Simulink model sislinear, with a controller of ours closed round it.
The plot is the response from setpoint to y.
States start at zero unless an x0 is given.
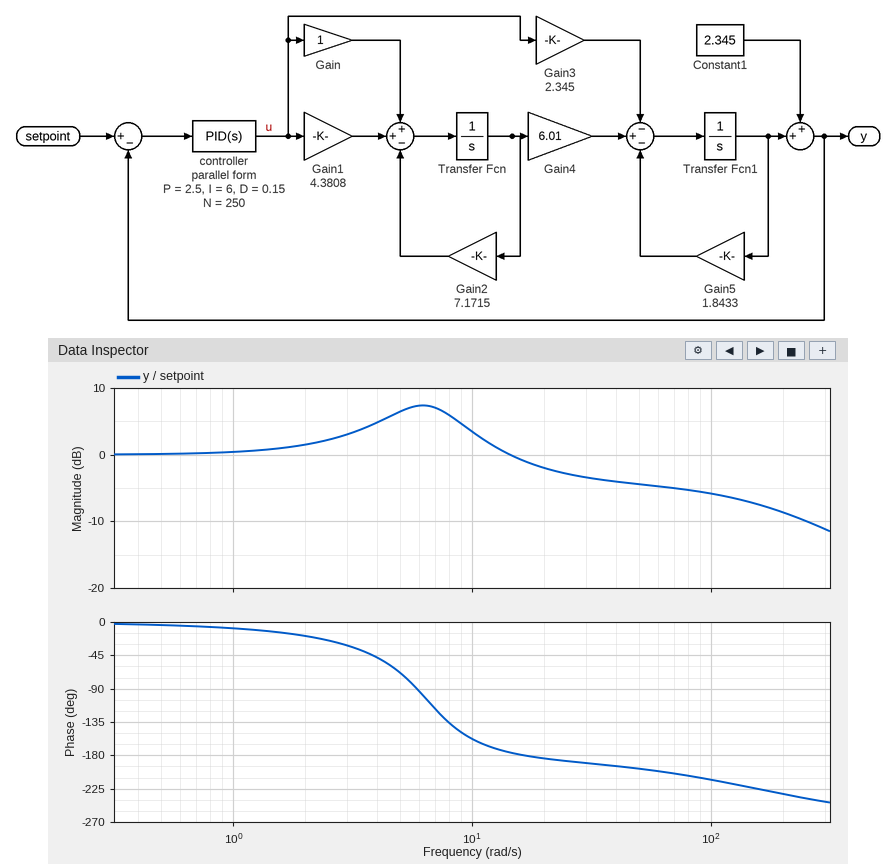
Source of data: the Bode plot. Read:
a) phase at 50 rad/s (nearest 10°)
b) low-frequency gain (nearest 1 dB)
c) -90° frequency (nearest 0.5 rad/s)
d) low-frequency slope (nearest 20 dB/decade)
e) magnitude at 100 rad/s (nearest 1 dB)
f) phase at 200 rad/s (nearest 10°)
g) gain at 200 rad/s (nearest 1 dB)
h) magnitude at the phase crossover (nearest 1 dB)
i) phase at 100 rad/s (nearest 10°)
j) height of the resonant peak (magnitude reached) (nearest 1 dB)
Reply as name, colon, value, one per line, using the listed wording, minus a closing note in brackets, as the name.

phase at 50 rad/s: -200°
low-frequency gain: 0 dB
-90° frequency: 6.0 rad/s
low-frequency slope: 0 dB/decade
magnitude at 100 rad/s: -6 dB
phase at 200 rad/s: -230°
gain at 200 rad/s: -9 dB
magnitude at the phase crossover: -1 dB
phase at 100 rad/s: -210°
height of the resonant peak (magnitude reached): 7 dB
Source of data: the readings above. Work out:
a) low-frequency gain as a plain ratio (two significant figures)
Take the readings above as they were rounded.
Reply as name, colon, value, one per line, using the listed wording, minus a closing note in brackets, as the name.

low-frequency gain as a plain ratio: 1.0
